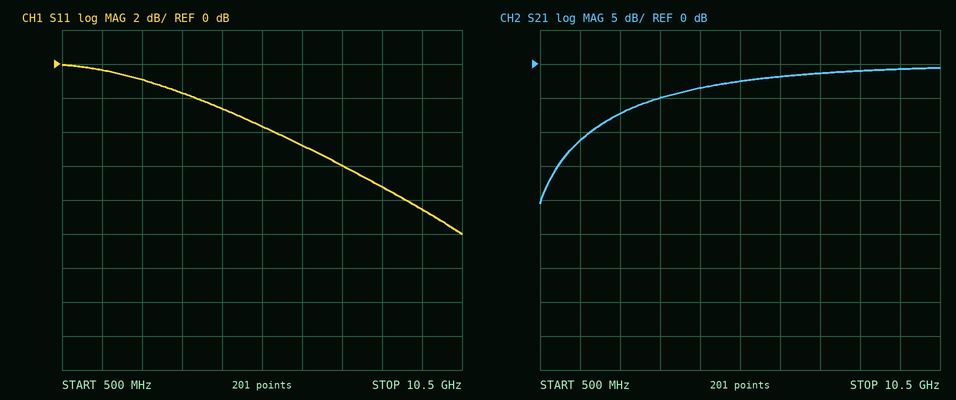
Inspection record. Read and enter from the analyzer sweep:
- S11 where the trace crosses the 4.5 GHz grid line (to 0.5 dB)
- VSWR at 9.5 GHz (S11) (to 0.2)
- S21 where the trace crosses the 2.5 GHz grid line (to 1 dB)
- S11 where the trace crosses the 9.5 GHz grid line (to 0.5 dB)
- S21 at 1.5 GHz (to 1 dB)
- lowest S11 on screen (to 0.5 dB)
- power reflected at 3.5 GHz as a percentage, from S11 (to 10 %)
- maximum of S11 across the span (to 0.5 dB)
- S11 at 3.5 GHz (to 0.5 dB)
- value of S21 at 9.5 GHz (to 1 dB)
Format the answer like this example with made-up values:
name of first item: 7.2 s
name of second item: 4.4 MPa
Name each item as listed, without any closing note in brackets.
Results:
S11 where the trace crosses the 4.5 GHz grid line: -2.5 dB
VSWR at 9.5 GHz (S11): 2.2
S21 where the trace crosses the 2.5 GHz grid line: -7 dB
S11 where the trace crosses the 9.5 GHz grid line: -8.5 dB
S21 at 1.5 GHz: -11 dB
lowest S11 on screen: -10.0 dB
power reflected at 3.5 GHz as a percentage, from S11: 70 %
maximum of S11 across the span: 0.0 dB
S11 at 3.5 GHz: -1.5 dB
value of S21 at 9.5 GHz: -1 dB
